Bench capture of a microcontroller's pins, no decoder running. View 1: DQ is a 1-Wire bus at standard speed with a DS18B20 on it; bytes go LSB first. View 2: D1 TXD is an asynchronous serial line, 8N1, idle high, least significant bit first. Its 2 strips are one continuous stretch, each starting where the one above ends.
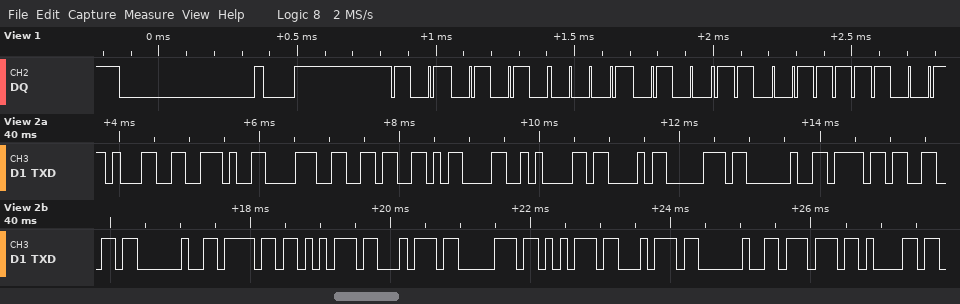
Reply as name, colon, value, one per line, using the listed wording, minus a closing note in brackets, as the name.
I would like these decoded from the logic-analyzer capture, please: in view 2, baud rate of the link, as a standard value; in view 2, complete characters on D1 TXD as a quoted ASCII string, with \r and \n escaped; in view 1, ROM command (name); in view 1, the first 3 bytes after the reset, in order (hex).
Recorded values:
in view 2, baud rate of the link, as a standard value: 9600 baud
in view 2, complete characters on D1 TXD as a quoted ASCII string, with \r and \n escaped: "1.86\r\nCp of output wa"
in view 1, ROM command: Match ROM
in view 1, the first 3 bytes after the reset, in order: 55 28 F3
